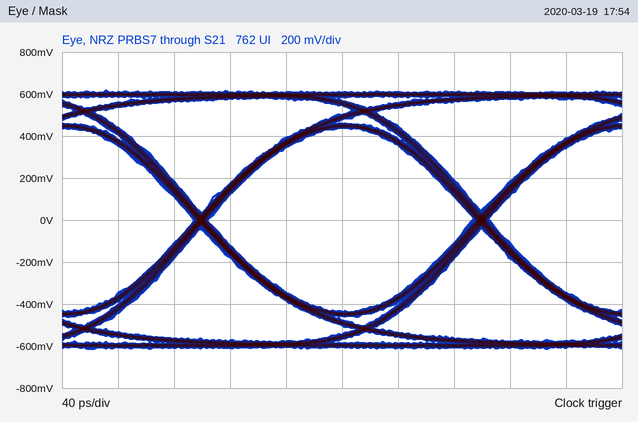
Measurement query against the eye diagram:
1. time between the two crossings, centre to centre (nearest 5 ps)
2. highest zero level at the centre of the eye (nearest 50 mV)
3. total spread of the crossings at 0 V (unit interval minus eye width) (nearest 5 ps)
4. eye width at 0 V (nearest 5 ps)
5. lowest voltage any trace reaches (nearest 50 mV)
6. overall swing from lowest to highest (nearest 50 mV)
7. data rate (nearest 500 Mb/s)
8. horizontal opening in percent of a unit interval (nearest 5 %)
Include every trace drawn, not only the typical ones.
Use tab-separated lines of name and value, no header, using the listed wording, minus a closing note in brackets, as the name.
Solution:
time between the two crossings, centre to centre	200 ps
highest zero level at the centre of the eye	-450 mV
total spread of the crossings at 0 V (unit interval minus eye width)	10 ps
eye width at 0 V	190 ps
lowest voltage any trace reaches	-600 mV
overall swing from lowest to highest	1.25 V
data rate	5.0 Gb/s
horizontal opening in percent of a unit interval	95 %
